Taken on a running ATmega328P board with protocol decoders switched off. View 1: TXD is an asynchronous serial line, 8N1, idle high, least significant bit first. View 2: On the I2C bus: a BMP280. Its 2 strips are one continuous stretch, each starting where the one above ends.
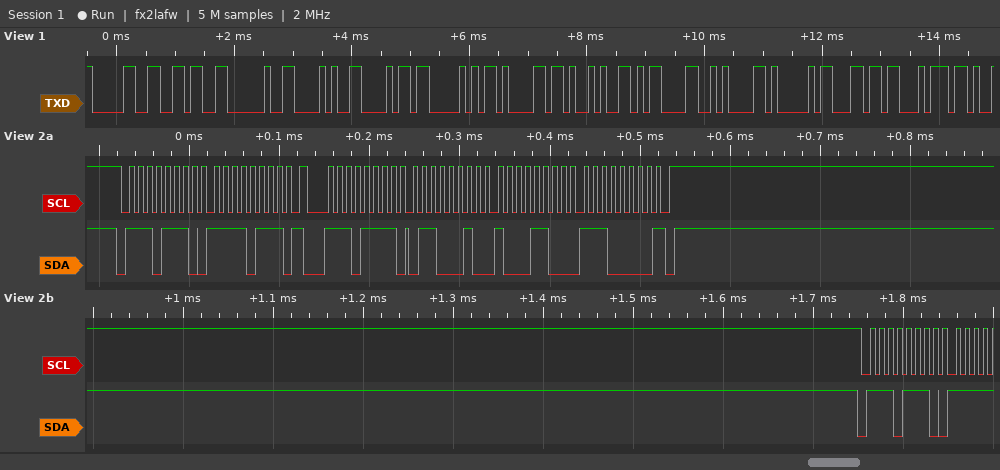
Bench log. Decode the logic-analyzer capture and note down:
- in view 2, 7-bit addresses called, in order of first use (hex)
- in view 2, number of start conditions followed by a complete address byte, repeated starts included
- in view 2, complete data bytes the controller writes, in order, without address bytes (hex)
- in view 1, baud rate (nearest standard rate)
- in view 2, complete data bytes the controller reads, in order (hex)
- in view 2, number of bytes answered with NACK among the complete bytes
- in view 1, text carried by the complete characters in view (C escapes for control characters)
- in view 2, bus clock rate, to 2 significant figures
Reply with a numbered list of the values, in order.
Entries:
1. 0x77
2. 3
3. F7
4. 9600 baud
5. 62 8C E0
6. 1
7. "06 (hPa)\r\nAlt"
8. 100 kHz
